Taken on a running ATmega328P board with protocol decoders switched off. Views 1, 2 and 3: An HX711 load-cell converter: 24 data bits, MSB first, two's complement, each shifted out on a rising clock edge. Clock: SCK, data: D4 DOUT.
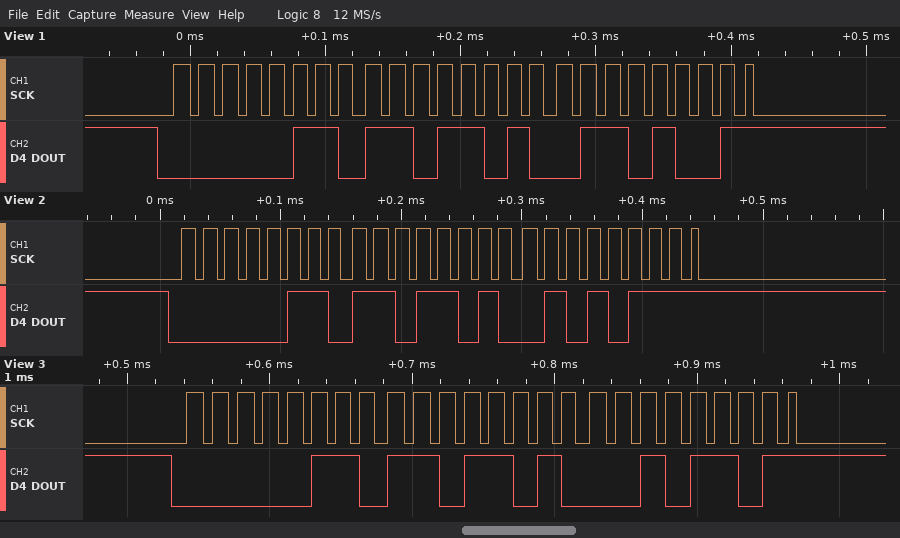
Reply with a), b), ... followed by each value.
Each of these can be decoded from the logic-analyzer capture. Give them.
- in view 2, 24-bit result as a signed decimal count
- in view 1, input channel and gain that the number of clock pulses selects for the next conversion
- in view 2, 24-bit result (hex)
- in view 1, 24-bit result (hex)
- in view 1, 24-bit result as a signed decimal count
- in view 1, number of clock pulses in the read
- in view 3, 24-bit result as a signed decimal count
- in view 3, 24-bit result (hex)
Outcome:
a) 449111
b) channel A, gain 128
c) 0x06DA57
d) 0x06DA69
e) 449129
f) 25
g) 449069
h) 0x06DA2D
